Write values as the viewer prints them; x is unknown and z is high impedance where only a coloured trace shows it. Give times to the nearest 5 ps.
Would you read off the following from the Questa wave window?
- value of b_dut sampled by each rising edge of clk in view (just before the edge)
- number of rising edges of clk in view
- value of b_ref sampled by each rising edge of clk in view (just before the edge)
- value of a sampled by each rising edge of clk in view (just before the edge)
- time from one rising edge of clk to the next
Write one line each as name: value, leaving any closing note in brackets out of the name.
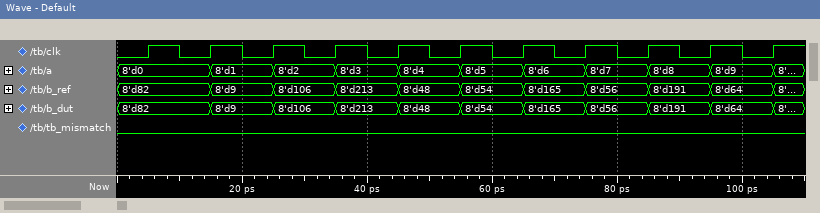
value of b_dut sampled by each rising edge of clk in view: 8'd82, 8'd82, 8'd9, 8'd106, 8'd213, 8'd48, 8'd54, 8'd165, 8'd56, 8'd191, 8'd64
number of rising edges of clk in view: 11
value of b_ref sampled by each rising edge of clk in view: 8'd82, 8'd82, 8'd9, 8'd106, 8'd213, 8'd48, 8'd54, 8'd165, 8'd56, 8'd191, 8'd64
value of a sampled by each rising edge of clk in view: 8'd0, 8'd0, 8'd1, 8'd2, 8'd3, 8'd4, 8'd5, 8'd6, 8'd7, 8'd8, 8'd9
time from one rising edge of clk to the next: 10 ps
